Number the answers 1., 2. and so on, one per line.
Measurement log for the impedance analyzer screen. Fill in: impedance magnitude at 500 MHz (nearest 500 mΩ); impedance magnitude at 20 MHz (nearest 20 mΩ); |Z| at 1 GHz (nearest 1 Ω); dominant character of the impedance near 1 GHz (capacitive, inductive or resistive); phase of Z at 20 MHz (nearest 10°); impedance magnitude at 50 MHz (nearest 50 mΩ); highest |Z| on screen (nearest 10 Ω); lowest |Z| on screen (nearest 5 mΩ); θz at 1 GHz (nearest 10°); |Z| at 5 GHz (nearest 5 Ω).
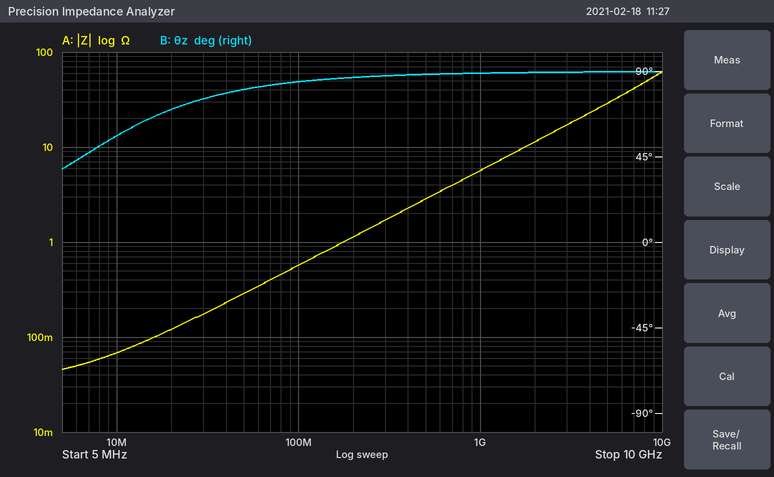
1. 3.0 Ω
2. 120 mΩ
3. 6 Ω
4. inductive
5. 70°
6. 300 mΩ
7. 60 Ω
8. 45 mΩ
9. 90°
10. 30 Ω
